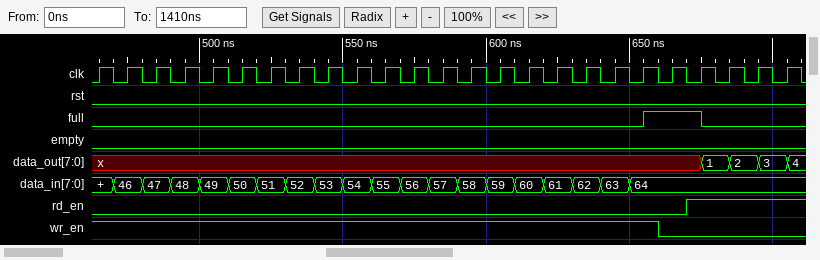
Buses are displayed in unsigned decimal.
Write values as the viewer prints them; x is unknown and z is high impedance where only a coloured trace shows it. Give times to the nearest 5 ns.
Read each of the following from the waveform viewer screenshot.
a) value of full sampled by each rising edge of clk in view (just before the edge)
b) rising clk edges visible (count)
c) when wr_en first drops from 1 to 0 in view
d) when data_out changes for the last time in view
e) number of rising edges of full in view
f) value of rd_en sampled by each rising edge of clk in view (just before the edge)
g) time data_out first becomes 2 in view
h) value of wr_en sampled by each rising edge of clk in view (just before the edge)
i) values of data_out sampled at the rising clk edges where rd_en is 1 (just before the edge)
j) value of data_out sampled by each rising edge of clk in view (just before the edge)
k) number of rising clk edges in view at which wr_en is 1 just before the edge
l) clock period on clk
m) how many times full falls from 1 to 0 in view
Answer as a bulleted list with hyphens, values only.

- 0 0 0 0 0 0 0 0 0 0 0 0 0 0 0 0 0 0 0 0 1 1 0 0 0
- 25
- 660 ns
- 705 ns
- 1
- 0 0 0 0 0 0 0 0 0 0 0 0 0 0 0 0 0 0 0 0 0 1 1 1 1
- 685 ns
- 1 1 1 1 1 1 1 1 1 1 1 1 1 1 1 1 1 1 1 1 0 0 0 0 0
- x, 1, 2, 3
- x, x, x, x, x, x, x, x, x, x, x, x, x, x, x, x, x, x, x, x, x, x, 1, 2, 3
- 20
- 10 ns
- 1
